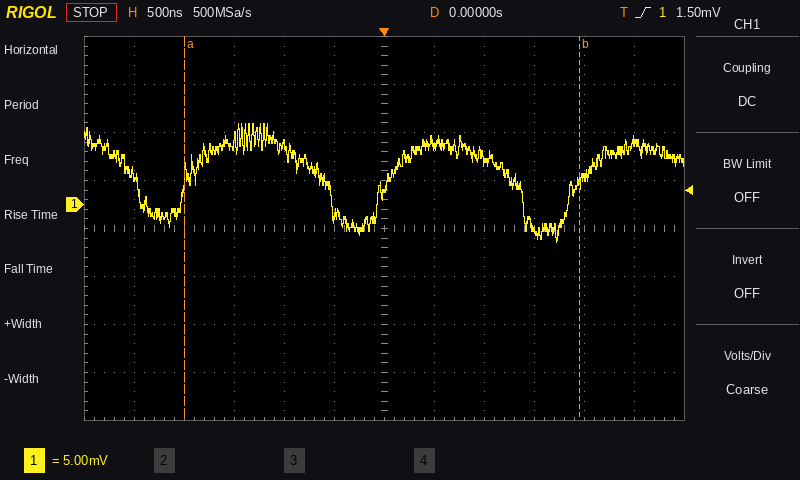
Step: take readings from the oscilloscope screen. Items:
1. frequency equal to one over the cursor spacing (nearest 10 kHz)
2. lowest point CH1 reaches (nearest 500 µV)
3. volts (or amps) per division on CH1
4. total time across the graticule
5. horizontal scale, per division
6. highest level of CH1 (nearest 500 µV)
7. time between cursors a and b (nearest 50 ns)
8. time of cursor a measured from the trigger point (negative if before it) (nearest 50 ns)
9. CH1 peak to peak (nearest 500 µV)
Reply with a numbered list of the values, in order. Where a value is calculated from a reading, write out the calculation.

1. 1 / 3.95 µs ≈ 250 kHz
2. -4.0 mV
3. 5 mV
4. 6 µs
5. 500 ns
6. 8.5 mV
7. 3.95 µs
8. -2.00 µs
9. 8.5 mV − (-4.0 mV) = 12.5 mV
